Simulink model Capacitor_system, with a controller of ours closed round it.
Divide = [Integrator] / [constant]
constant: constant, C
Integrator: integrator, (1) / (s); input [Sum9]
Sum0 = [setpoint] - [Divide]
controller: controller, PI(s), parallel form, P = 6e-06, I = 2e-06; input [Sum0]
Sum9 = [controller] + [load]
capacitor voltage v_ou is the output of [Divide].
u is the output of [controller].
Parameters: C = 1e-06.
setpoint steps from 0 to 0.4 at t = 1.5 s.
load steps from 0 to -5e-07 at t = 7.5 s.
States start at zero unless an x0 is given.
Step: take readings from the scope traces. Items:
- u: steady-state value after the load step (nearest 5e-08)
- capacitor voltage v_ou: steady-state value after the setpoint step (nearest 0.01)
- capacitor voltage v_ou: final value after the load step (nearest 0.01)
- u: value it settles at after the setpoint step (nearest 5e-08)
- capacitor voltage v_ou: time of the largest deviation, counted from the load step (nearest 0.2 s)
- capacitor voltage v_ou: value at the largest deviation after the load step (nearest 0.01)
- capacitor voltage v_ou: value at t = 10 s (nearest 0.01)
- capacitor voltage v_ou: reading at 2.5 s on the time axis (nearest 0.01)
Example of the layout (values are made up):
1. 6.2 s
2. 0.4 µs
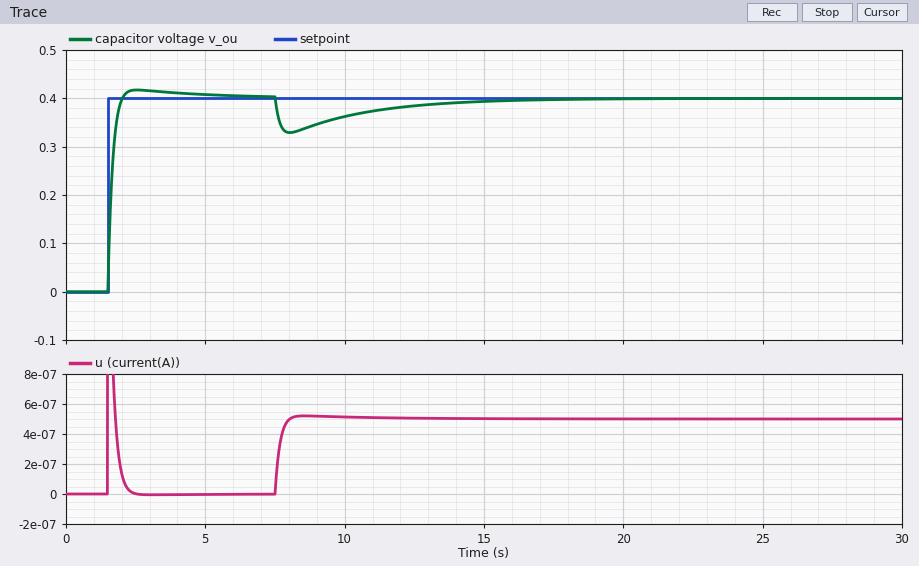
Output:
1. 0.00000050
2. 0.40
3. 0.40
4. 0.00000000
5. 0.6 s
6. 0.33
7. 0.36
8. 0.42
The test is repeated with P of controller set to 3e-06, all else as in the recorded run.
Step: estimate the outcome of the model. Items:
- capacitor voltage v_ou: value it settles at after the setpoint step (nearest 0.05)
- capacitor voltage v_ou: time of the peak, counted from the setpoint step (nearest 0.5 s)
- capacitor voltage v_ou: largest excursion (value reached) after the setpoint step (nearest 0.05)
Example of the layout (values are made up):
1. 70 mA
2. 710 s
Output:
1. 0.40
2. 1.5 s
3. 0.45
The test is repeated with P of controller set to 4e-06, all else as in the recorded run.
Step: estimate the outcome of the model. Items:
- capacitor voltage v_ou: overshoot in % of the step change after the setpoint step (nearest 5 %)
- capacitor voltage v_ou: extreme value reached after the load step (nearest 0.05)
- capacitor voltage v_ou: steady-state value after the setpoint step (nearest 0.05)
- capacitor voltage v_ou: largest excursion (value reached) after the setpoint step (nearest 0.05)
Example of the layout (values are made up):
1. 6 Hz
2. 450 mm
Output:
1. 10 %
2. 0.30
3. 0.40
4. 0.45
